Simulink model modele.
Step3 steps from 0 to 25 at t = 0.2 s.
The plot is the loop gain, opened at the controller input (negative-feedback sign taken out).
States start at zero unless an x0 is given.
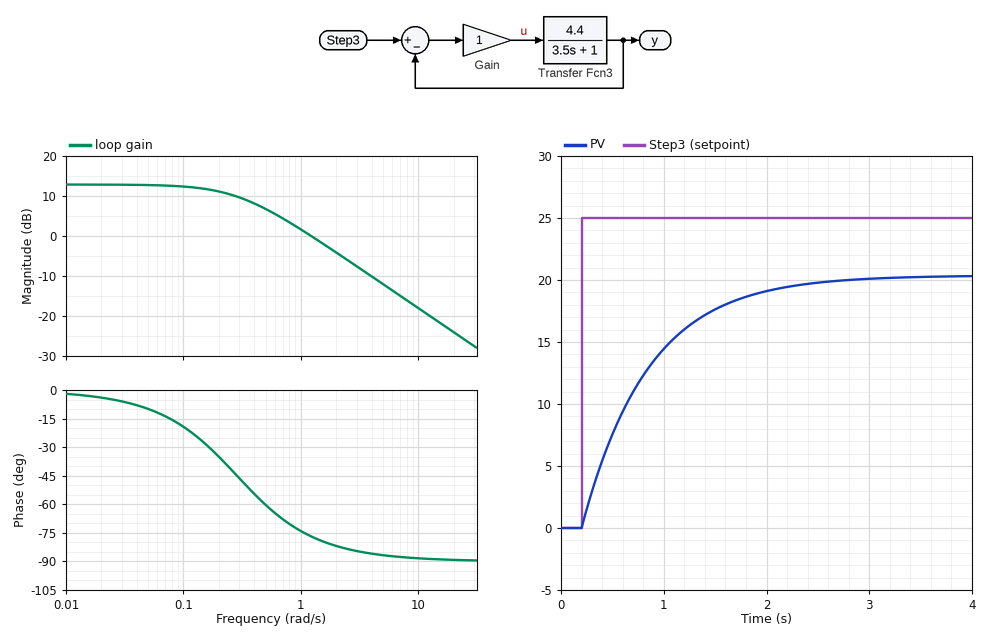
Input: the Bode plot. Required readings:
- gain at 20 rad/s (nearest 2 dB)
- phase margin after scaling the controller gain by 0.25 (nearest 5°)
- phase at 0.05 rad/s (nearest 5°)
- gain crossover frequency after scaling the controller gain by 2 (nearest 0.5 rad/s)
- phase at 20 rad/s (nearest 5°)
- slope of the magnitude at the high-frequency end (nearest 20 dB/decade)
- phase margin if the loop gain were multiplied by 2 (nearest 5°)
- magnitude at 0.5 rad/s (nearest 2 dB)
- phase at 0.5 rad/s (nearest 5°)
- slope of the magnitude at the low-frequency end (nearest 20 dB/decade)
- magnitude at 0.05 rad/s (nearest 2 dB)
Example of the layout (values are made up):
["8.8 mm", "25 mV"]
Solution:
["-24 dB", "155°", "-10°", "2.5 rad/s", "-90°", "-20 dB/decade", "95°", "6 dB", "-60°", "0 dB/decade", "12 dB"]
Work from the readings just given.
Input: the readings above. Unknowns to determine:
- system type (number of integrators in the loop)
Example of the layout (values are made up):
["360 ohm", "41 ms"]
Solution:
["0"]
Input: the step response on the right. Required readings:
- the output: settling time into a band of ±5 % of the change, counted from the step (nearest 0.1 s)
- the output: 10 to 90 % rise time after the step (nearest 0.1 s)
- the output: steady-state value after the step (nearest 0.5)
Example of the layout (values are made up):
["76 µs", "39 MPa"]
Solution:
["1.9 s", "1.4 s", "20.5"]
